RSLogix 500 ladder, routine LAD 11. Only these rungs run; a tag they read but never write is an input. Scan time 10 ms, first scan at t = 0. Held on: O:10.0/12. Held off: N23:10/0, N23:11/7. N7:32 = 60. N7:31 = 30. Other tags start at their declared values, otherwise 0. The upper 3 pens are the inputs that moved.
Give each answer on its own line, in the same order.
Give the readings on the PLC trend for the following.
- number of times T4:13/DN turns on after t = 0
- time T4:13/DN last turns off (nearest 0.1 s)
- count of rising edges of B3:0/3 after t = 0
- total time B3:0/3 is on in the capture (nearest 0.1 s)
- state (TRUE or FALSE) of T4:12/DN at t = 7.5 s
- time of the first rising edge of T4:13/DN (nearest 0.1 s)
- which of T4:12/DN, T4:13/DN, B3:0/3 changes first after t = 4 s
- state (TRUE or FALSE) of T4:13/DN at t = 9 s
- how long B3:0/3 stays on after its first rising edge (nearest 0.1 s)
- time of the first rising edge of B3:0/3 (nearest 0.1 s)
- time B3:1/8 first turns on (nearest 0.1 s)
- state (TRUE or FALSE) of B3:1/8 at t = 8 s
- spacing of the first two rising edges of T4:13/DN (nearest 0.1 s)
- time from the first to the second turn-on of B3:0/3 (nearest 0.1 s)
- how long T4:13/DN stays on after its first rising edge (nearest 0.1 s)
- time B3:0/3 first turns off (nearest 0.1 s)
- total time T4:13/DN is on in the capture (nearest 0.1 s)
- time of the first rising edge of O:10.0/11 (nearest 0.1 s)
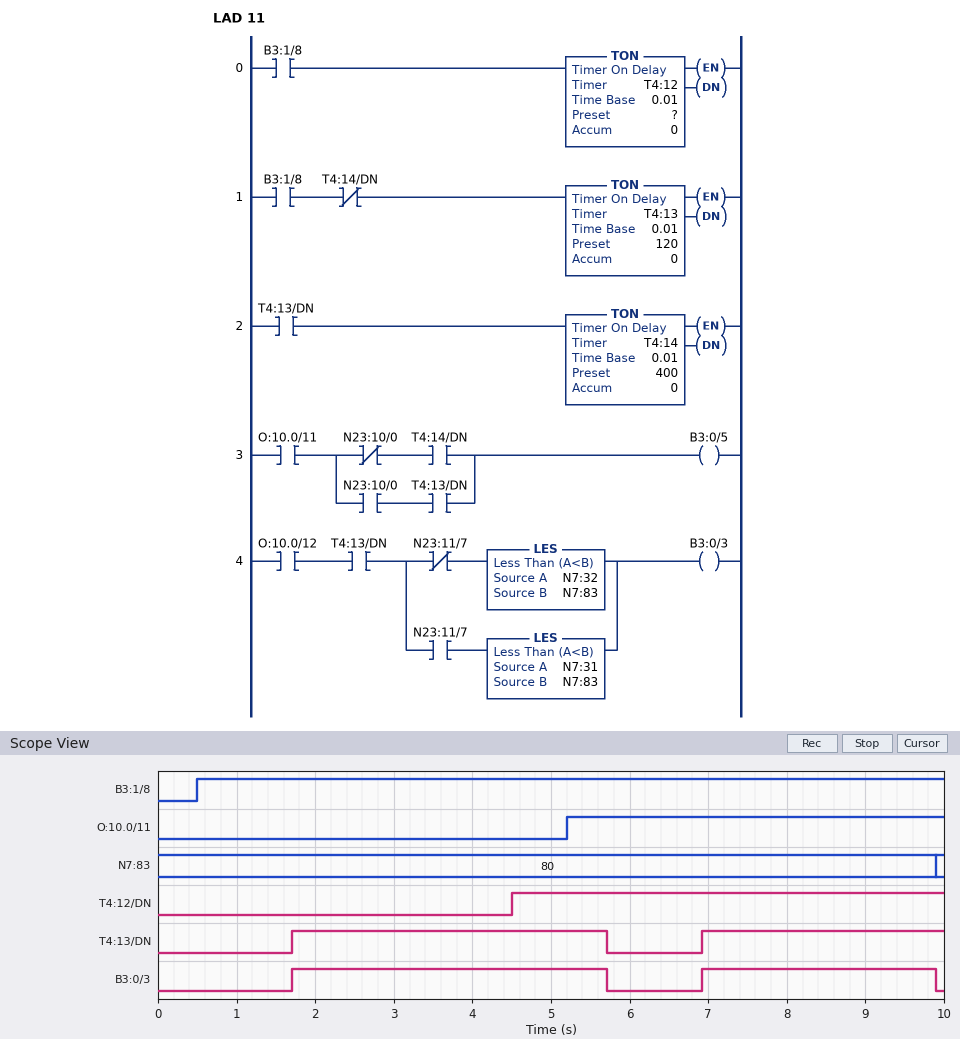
2
5.7 s
2
7.0 s
TRUE
1.7 s
T4:12/DN
TRUE
4.0 s
1.7 s
0.5 s
TRUE
5.2 s
5.2 s
4.0 s
5.7 s
7.1 s
5.2 s
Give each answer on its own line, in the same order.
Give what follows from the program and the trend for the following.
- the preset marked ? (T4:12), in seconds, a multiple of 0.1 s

4.0 s
